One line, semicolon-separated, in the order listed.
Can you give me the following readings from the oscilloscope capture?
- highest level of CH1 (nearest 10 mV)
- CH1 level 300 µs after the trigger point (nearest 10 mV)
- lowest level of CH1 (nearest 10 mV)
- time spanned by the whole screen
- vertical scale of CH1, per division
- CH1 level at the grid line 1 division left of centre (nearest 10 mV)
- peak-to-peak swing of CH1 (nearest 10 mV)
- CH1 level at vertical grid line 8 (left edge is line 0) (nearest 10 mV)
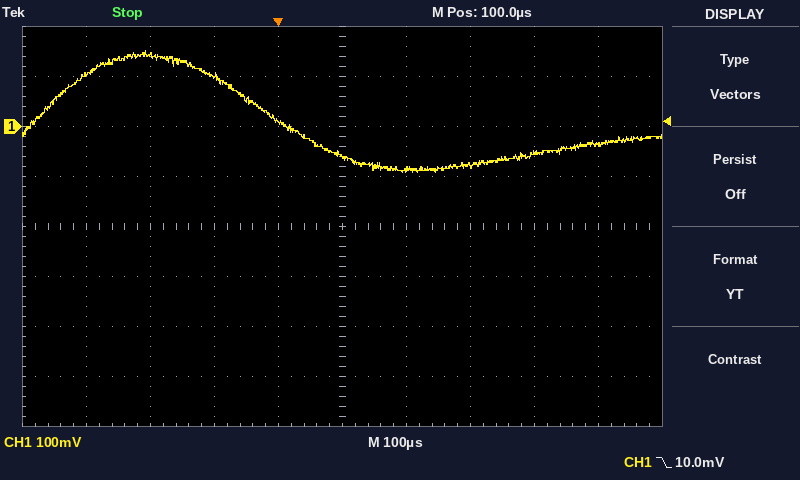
150 mV; -80 mV; -90 mV; 1 ms; 100 mV; 10 mV; 240 mV; -50 mV
